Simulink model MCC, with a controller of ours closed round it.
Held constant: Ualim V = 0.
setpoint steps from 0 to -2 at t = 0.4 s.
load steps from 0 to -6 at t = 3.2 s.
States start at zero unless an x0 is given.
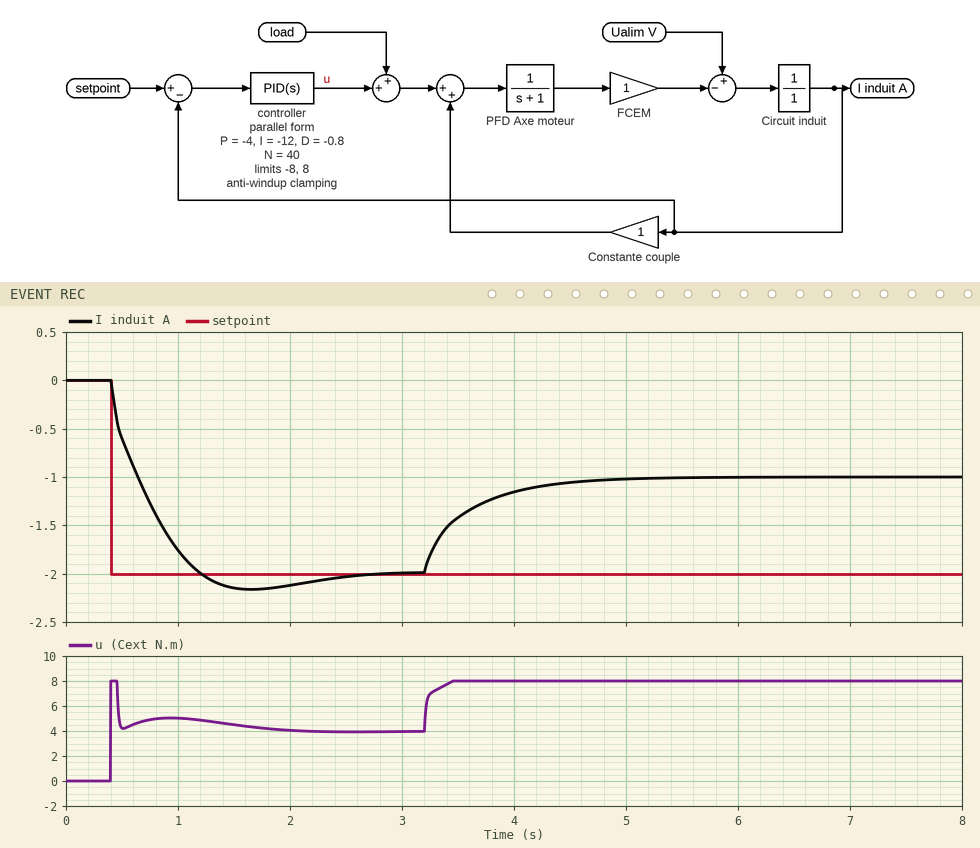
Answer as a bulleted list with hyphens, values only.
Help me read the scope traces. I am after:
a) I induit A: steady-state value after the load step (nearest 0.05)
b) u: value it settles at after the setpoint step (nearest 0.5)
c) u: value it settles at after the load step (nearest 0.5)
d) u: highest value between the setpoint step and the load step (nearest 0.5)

- -1.00
- 4.0
- 8.0
- 8.0
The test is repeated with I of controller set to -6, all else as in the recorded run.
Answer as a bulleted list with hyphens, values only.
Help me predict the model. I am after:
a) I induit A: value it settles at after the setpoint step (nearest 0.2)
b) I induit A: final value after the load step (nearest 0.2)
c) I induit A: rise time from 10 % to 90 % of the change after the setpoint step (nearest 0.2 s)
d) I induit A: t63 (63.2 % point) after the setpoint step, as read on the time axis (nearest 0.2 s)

- -2.0
- -1.0
- 1.0 s
- 0.8 s
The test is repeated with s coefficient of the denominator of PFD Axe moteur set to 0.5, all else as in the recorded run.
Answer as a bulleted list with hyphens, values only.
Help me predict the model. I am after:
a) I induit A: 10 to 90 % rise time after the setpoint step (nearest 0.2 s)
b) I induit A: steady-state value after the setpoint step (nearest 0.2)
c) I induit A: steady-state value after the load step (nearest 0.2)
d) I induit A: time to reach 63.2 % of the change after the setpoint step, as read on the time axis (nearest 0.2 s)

- 0.6 s
- -2.0
- -1.0
- 0.6 s
